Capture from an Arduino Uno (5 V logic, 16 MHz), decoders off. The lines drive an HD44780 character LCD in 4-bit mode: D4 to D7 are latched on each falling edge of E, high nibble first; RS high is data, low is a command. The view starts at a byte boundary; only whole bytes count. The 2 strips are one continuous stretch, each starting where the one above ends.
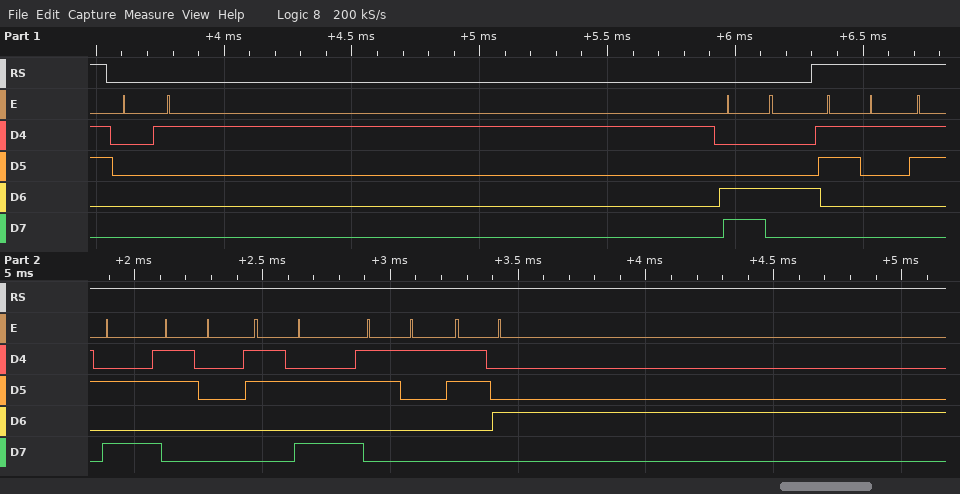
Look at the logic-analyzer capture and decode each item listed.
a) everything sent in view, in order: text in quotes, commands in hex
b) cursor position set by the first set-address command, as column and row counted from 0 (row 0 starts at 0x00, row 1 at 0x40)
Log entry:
0x01 0xC4 "1:0:14"
column 4, row 1
